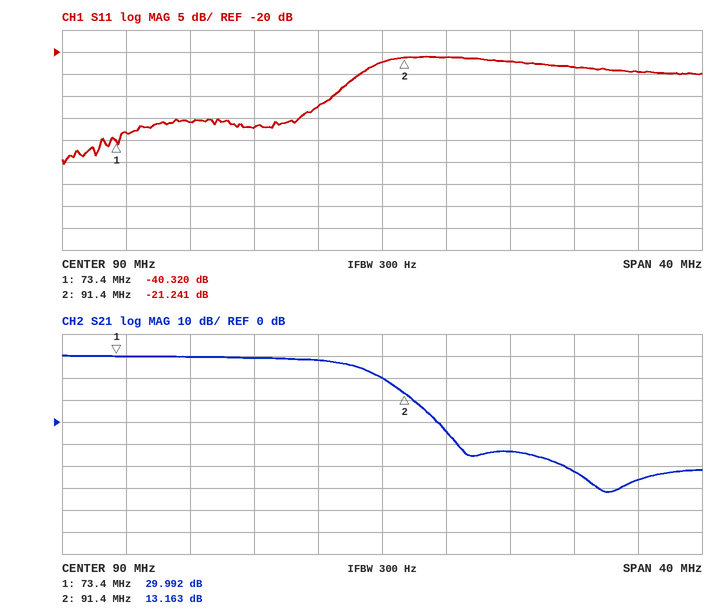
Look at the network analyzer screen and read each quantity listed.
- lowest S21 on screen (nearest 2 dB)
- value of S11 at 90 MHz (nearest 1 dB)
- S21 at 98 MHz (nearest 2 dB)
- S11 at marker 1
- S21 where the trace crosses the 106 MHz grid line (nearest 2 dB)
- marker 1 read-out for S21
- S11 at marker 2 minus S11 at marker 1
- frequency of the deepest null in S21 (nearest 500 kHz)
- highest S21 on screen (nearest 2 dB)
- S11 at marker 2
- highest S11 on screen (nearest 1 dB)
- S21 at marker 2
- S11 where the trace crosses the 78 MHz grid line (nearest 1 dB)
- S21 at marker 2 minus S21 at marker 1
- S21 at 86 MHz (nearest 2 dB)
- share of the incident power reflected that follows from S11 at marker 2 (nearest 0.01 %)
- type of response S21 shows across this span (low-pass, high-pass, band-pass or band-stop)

-32 dB
-22 dB
-14 dB
-40.320 dB
-26 dB
29.992 dB
19.079 dB
104.0 MHz
30 dB
-21.241 dB
-21 dB
13.163 dB
-36 dB
-16.829 dB
28 dB
0.75 %
low-pass
